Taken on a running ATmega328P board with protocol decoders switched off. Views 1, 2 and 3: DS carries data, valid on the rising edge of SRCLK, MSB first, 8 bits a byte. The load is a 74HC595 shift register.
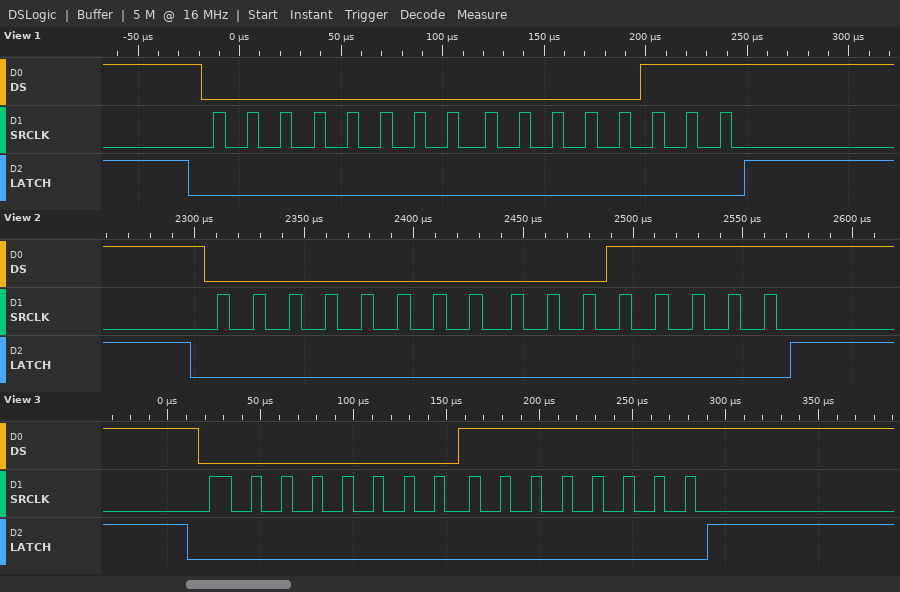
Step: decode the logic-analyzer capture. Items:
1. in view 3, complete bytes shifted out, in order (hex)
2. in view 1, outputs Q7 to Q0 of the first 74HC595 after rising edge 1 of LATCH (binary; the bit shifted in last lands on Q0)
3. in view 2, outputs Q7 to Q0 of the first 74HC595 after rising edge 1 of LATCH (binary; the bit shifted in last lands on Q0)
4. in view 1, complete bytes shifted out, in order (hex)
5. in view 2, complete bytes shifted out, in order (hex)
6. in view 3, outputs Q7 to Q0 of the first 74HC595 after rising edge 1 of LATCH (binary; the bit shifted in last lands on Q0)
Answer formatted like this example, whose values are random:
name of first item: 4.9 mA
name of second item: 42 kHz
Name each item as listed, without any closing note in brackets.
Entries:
in view 3, complete bytes shifted out, in order: 0x00 0xFF
in view 1, outputs Q7 to Q0 of the first 74HC595 after rising edge 1 of LATCH: 00000111
in view 2, outputs Q7 to Q0 of the first 74HC595 after rising edge 1 of LATCH: 00011111
in view 1, complete bytes shifted out, in order: 0x00 0x07
in view 2, complete bytes shifted out, in order: 00 1F
in view 3, outputs Q7 to Q0 of the first 74HC595 after rising edge 1 of LATCH: 11111111
